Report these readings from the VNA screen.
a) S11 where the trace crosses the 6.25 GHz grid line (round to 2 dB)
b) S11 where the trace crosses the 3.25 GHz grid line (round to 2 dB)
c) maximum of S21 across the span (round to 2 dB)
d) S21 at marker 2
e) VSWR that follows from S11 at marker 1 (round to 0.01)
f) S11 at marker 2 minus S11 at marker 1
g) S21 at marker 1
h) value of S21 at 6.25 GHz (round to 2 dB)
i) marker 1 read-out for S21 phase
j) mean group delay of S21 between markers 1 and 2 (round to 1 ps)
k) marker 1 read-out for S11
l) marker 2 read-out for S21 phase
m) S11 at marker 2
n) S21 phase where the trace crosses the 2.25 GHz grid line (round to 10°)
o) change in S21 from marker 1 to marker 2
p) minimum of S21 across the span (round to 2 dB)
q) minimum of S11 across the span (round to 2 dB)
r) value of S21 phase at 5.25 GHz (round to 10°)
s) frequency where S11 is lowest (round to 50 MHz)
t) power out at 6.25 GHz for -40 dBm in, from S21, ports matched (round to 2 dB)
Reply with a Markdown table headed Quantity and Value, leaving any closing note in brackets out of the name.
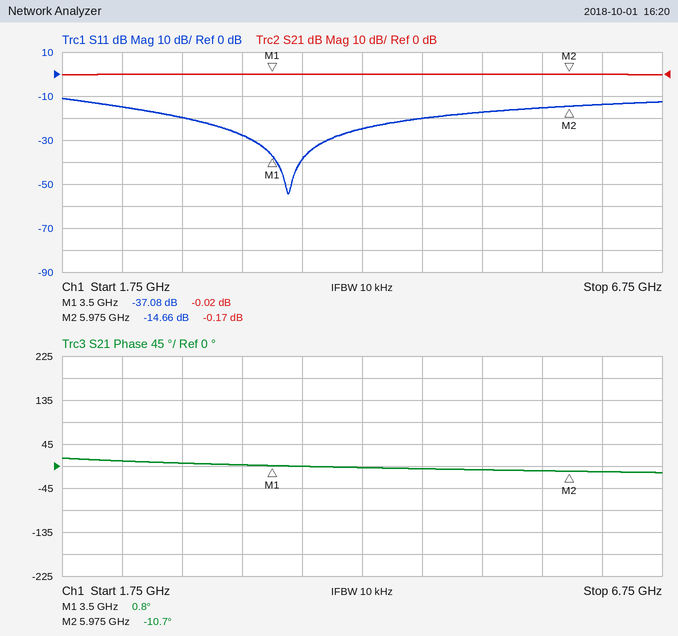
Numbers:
| Quantity | Value |
|---|---|
| S11 where the trace crosses the 6.25 GHz grid line | -14 dB |
| S11 where the trace crosses the 3.25 GHz grid line | -28 dB |
| maximum of S21 across the span | 0 dB |
| S21 at marker 2 | -0.17 dB |
| VSWR that follows from S11 at marker 1 | 1.03 |
| S11 at marker 2 minus S11 at marker 1 | 22.42 dB |
| S21 at marker 1 | -0.02 dB |
| value of S21 at 6.25 GHz | 0 dB |
| marker 1 read-out for S21 phase | 0.8° |
| mean group delay of S21 between markers 1 and 2 | 13 ps |
| marker 1 read-out for S11 | -37.08 dB |
| marker 2 read-out for S21 phase | -10.7° |
| S11 at marker 2 | -14.66 dB |
| S21 phase where the trace crosses the 2.25 GHz grid line | 10° |
| change in S21 from marker 1 to marker 2 | -0.15 dB |
| minimum of S21 across the span | 0 dB |
| minimum of S11 across the span | -54 dB |
| value of S21 phase at 5.25 GHz | -10° |
| frequency where S11 is lowest | 3.65 GHz |
| power out at 6.25 GHz for -40 dBm in, from S21, ports matched | -40 dBm |
